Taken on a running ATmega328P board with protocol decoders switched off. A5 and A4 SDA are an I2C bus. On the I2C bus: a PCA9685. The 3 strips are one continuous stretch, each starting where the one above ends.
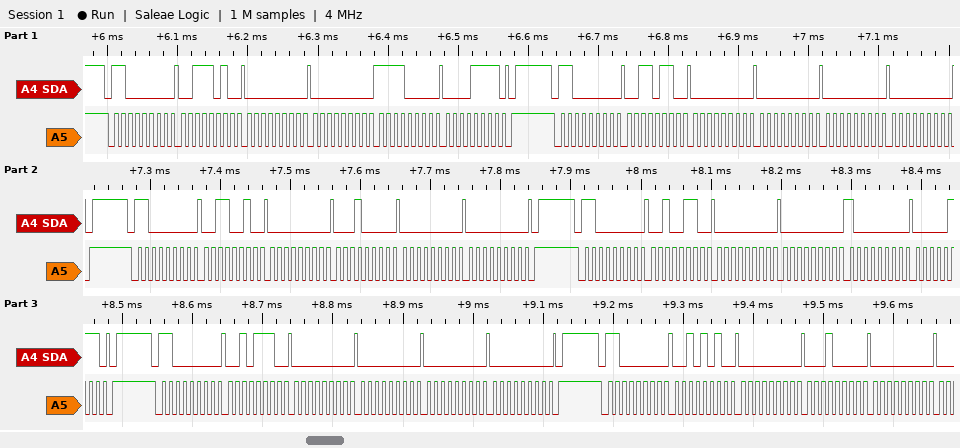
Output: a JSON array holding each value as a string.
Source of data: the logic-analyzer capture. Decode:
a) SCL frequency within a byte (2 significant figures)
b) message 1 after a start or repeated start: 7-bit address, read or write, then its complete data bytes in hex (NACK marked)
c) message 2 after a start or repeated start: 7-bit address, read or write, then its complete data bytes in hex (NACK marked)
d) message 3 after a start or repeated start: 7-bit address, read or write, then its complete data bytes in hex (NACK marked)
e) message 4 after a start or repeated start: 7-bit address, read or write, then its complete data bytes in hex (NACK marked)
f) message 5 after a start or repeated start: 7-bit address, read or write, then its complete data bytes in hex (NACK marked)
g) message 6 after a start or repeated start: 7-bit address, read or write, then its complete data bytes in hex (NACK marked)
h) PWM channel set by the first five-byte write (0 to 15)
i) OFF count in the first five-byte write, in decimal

["100 kHz", "0x60 write: 3A 00 00 F0 0F", "0x60 write: 36 00 00 00 00", "0x60 write: 32 00 10 00 00", "0x60 write: 26 00 00 80 07", "0x60 write: 2E 00 00 00 00", "0x60 write: 2A 00 10 00", "13", "4080"]
